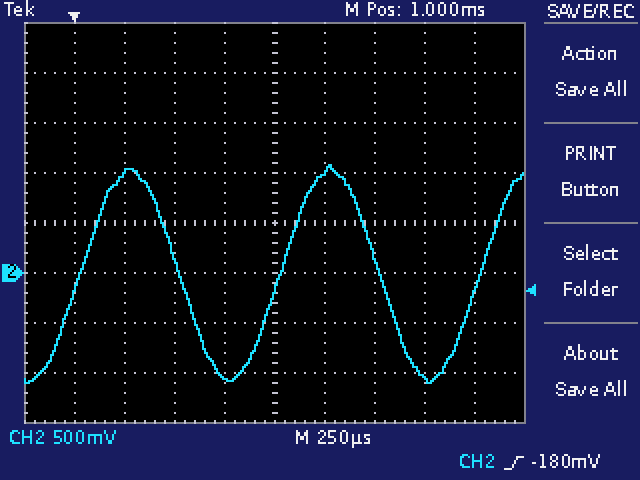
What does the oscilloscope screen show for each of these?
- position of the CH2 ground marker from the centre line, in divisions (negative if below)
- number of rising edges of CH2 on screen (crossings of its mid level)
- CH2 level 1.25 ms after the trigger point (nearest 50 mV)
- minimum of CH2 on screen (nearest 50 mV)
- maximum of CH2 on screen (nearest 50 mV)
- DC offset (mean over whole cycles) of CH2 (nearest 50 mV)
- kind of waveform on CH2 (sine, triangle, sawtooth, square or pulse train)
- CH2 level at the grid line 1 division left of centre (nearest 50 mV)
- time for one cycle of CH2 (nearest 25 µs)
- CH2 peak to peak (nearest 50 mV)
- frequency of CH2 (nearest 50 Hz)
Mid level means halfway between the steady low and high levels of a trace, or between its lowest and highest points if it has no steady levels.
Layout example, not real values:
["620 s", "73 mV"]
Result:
["-1.0 div", "3", "1.00 V", "-1.10 V", "1.10 V", "0 mV", "sine", "-1.05 V", "1.000 ms", "2.20 V", "1.00 kHz"]
